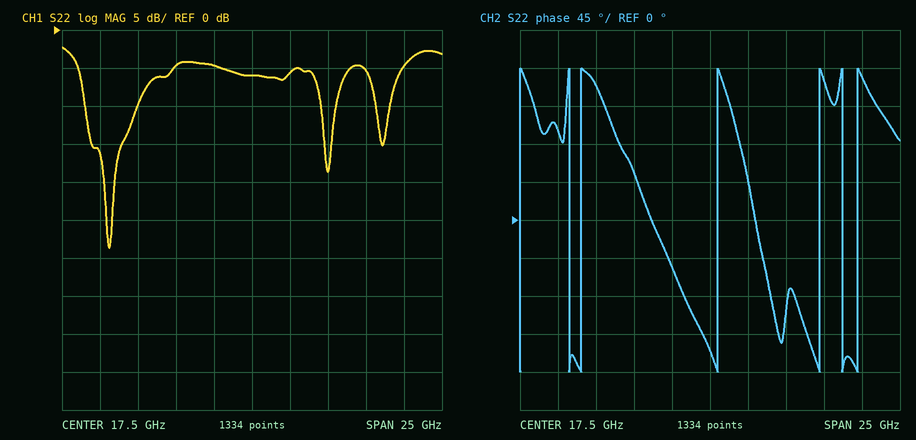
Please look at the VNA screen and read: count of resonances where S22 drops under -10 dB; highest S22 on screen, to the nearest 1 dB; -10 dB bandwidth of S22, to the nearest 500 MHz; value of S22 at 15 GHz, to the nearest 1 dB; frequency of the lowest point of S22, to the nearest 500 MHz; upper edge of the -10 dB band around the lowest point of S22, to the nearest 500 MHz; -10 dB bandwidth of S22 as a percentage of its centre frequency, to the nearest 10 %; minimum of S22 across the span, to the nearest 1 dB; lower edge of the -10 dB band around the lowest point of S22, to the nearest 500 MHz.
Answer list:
3
-2 dB
3.5 GHz
-5 dB
8.0 GHz
10.0 GHz
40 %
-29 dB
6.5 GHz
